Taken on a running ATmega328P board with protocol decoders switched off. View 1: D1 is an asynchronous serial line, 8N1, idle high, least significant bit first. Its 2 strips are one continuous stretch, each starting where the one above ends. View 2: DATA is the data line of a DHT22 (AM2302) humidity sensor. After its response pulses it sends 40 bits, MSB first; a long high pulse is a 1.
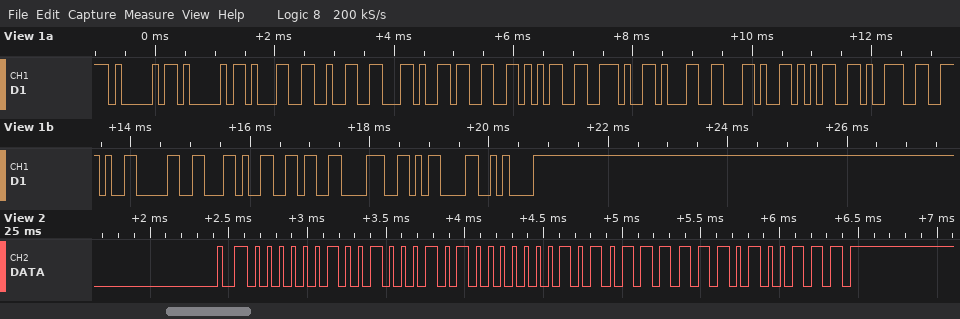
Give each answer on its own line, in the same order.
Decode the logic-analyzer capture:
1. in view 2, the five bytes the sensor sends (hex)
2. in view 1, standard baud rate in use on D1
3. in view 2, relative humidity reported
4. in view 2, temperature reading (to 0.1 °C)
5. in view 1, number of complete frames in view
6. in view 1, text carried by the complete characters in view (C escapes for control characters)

02 45 01 5F A7
9600 baud
58.1 %
35.1 °C
19
"AA12,35.1,59.0,68\r\n"
